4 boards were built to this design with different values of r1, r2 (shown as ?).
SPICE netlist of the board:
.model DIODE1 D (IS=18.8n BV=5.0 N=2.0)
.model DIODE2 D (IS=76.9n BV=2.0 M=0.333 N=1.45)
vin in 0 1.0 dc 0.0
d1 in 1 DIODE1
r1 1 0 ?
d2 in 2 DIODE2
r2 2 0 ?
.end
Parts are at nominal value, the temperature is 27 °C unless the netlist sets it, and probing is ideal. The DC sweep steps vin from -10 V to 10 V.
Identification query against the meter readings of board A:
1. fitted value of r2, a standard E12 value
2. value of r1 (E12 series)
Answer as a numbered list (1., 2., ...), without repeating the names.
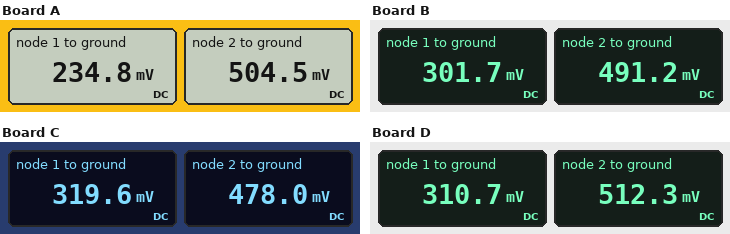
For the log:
1. 12 Ω
2. 4.7 Ω
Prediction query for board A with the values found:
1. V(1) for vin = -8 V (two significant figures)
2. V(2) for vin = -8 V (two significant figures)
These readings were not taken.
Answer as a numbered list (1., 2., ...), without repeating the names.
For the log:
1. -2.7 V
2. -5.8 V
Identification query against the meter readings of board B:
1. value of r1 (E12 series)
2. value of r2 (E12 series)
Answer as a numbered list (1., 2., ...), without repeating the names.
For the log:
1. 22 Ω
2. 8.2 Ω
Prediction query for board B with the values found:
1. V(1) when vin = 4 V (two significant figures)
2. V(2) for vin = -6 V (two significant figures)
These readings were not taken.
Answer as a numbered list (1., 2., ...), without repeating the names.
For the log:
1. 3.2 V
2. -3.8 V
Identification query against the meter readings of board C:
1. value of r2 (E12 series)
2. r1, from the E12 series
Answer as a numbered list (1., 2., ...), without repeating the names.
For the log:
1. 5.6 Ω
2. 33 Ω
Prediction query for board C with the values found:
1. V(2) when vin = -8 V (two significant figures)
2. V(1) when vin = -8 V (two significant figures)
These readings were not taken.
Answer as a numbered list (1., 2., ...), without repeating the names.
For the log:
1. -5.7 V
2. -2.8 V
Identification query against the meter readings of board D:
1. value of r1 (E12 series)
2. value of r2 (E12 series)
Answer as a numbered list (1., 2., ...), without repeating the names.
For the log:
1. 27 Ω
2. 15 Ω
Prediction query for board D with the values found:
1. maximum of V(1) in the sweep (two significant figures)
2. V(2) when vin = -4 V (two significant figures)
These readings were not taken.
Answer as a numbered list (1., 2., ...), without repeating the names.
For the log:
1. 9.1 V
2. -1.8 V
